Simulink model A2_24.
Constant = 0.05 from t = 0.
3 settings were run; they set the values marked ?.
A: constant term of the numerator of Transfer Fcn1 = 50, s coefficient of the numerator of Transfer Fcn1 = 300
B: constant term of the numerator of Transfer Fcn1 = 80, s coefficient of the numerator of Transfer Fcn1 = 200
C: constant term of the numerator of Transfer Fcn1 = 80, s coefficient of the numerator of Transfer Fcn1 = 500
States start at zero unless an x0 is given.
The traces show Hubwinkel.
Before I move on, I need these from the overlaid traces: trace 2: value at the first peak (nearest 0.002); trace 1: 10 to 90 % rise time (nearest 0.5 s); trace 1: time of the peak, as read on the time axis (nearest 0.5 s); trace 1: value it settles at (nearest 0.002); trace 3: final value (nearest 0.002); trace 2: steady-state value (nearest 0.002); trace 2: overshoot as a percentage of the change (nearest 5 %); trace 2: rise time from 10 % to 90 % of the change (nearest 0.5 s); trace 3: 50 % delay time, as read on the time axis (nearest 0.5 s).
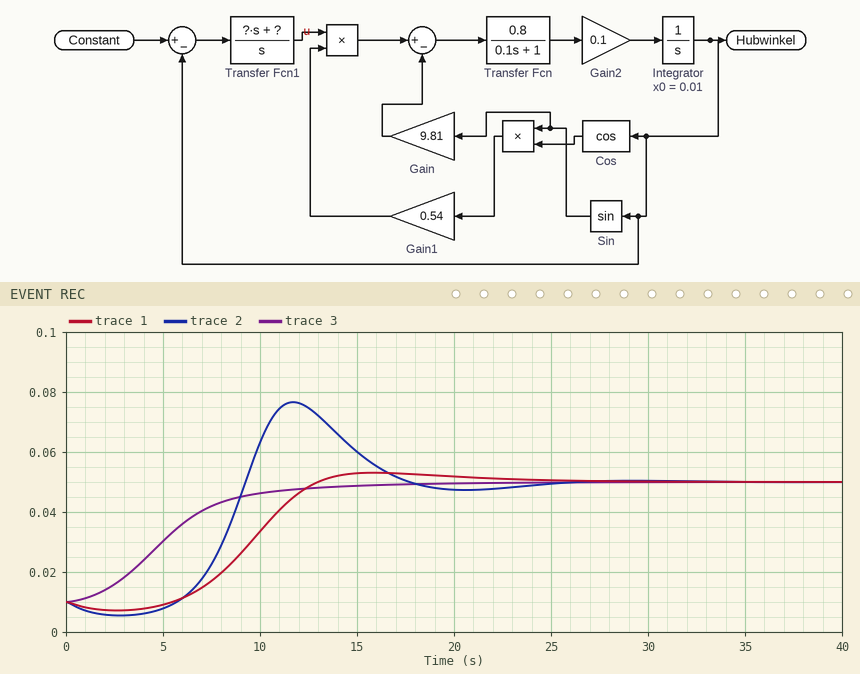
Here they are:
0.076
5.0 s
16.0 s
0.050
0.050
0.050
65 %
2.5 s
5.0 s
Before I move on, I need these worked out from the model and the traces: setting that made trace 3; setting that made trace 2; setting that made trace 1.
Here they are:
C
B
A
